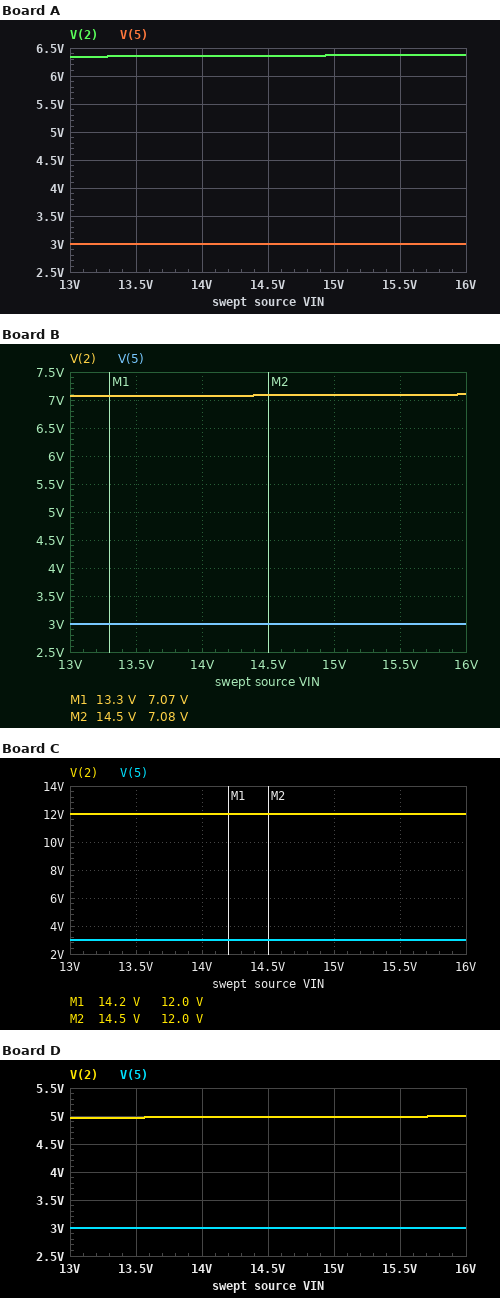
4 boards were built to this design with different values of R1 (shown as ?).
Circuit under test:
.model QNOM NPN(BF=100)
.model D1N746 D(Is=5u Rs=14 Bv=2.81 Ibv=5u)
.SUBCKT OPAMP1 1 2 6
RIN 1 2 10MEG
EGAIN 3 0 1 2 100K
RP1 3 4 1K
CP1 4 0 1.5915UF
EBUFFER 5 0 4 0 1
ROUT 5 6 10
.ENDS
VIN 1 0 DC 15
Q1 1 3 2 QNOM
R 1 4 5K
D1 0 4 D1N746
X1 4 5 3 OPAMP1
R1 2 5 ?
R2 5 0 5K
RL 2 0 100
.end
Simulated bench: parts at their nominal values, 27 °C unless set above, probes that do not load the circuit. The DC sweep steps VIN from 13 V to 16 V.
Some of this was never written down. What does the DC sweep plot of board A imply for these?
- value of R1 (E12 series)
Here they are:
5.6 kΩ
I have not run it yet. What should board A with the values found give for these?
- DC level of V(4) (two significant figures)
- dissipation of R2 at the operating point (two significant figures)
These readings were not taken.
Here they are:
3.0 V
1.8 mW
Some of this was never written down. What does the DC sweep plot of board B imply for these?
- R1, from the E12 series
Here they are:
6.8 kΩ
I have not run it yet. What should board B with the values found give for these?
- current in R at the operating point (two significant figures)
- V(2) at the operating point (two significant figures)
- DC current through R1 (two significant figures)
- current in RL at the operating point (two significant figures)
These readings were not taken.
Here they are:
2.4 mA
7.1 V
600 µA
71 mA
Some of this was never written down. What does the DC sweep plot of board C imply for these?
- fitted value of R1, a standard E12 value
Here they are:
15 kΩ
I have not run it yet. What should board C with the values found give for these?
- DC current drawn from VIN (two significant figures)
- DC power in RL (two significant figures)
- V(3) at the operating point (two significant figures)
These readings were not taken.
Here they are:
120 mA
1.4 W
13 V
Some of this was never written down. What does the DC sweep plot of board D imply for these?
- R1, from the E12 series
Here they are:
3.3 kΩ
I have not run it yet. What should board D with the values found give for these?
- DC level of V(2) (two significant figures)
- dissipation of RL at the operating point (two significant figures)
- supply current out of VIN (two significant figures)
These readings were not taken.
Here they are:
5.0 V
250 mW
52 mA
